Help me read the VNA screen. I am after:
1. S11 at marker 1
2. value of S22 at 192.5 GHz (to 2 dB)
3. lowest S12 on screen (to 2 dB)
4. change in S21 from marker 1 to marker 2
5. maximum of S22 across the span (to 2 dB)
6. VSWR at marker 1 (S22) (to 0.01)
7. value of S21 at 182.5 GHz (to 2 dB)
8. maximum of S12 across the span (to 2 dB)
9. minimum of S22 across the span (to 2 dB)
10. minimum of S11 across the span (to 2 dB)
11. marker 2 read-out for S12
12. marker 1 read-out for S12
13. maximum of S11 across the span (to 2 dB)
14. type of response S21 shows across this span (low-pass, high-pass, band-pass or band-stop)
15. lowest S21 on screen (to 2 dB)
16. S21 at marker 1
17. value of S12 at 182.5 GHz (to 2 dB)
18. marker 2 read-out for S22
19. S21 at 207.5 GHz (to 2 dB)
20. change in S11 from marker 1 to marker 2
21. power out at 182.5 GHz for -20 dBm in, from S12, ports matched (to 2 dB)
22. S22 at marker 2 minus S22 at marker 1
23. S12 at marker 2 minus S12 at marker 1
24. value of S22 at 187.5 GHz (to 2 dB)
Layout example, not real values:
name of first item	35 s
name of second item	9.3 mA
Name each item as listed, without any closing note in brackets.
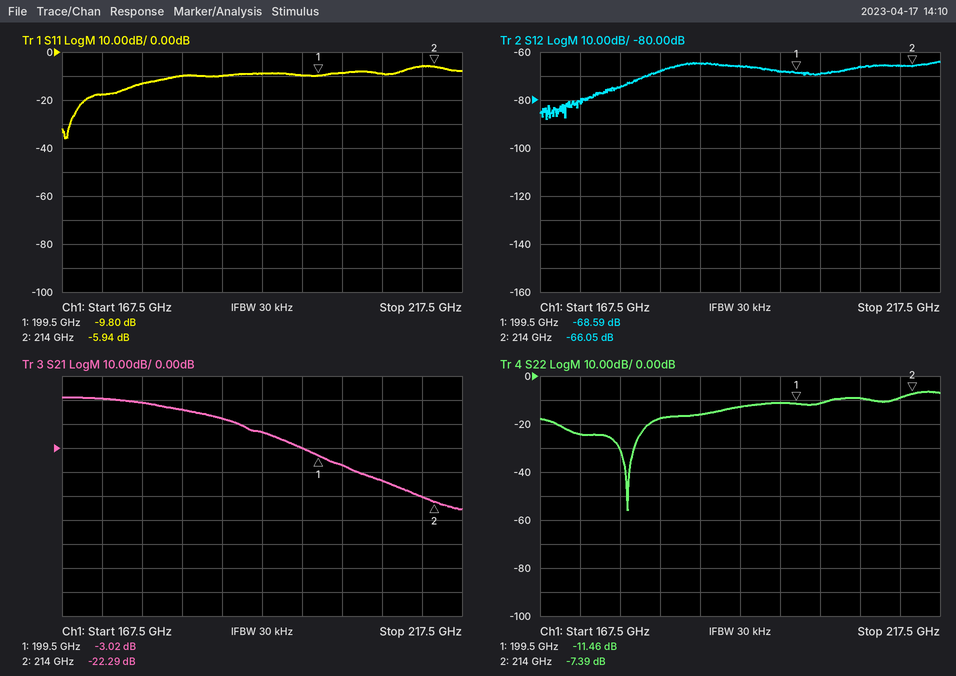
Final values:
S11 at marker 1	-9.80 dB
value of S22 at 192.5 GHz	-12 dB
lowest S12 on screen	-88 dB
change in S21 from marker 1 to marker 2	-19.27 dB
maximum of S22 across the span	-6 dB
VSWR at marker 1 (S22)	1.73
value of S21 at 182.5 GHz	16 dB
maximum of S12 across the span	-64 dB
minimum of S22 across the span	-56 dB
minimum of S11 across the span	-36 dB
marker 2 read-out for S12	-66.05 dB
marker 1 read-out for S12	-68.59 dB
maximum of S11 across the span	-6 dB
type of response S21 shows across this span	low-pass
lowest S21 on screen	-26 dB
S21 at marker 1	-3.02 dB
value of S12 at 182.5 GHz	-68 dB
marker 2 read-out for S22	-7.39 dB
S21 at 207.5 GHz	-14 dB
change in S11 from marker 1 to marker 2	3.86 dB
power out at 182.5 GHz for -20 dBm in, from S12, ports matched	-88 dBm
S22 at marker 2 minus S22 at marker 1	4.07 dB
S12 at marker 2 minus S12 at marker 1	2.54 dB
value of S22 at 187.5 GHz	-16 dB
